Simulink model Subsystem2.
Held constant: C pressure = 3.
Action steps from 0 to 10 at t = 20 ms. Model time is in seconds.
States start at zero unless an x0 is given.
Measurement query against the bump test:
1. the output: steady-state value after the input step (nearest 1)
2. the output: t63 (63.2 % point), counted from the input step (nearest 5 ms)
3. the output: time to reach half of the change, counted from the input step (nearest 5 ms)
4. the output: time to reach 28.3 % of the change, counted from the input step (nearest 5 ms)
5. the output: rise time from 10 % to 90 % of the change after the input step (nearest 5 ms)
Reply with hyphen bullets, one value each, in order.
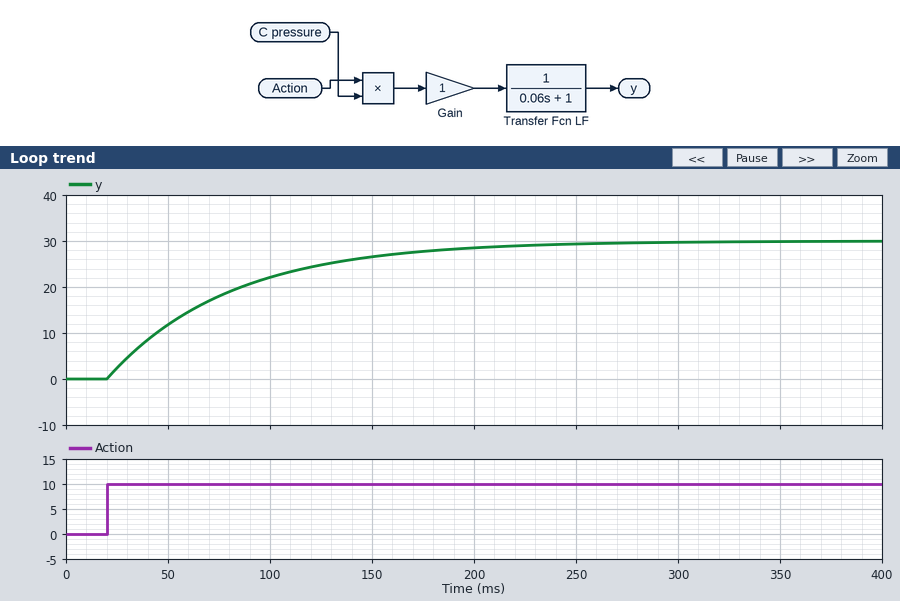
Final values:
- 30
- 60 ms
- 40 ms
- 20 ms
- 130 ms
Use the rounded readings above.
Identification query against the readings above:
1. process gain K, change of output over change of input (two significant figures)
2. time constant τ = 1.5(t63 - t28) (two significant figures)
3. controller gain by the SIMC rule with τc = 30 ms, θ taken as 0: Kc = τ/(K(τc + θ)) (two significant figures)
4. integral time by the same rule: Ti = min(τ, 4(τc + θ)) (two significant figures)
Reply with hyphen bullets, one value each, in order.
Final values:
- 3.0
- 60 ms
- 0.67
- 60 ms
